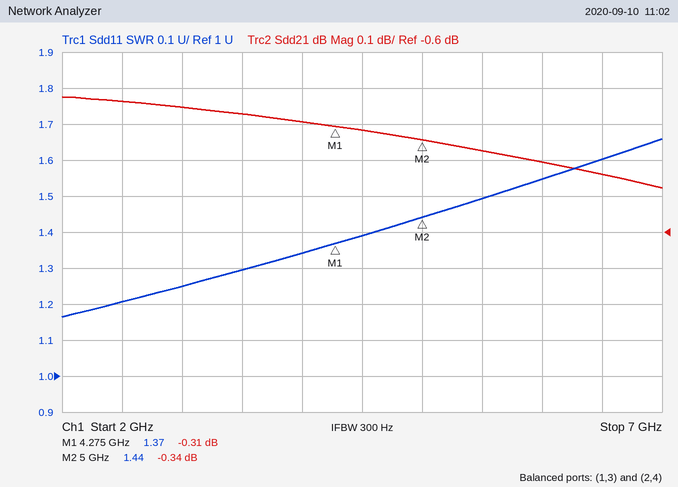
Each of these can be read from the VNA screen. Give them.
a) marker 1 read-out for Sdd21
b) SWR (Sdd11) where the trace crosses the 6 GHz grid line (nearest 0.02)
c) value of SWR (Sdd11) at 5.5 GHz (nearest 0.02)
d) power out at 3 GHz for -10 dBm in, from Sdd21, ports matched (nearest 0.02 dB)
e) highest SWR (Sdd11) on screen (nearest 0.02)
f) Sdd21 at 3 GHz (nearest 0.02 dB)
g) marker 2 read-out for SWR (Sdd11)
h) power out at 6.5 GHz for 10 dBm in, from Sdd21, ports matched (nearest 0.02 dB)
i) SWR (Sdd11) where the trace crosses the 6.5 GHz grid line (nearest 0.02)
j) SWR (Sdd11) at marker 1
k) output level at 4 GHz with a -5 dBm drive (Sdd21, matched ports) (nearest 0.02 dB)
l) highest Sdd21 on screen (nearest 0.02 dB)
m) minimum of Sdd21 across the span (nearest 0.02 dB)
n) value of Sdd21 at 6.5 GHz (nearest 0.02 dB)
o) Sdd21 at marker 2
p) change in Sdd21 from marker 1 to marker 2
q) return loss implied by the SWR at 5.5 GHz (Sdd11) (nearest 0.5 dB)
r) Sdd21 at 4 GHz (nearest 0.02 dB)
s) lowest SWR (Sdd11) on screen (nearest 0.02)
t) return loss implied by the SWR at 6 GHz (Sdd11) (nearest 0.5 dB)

-0.31 dB
1.54
1.50
-10.26 dBm
1.66
-0.26 dB
1.44
9.56 dBm
1.60
1.37
-5.30 dBm
-0.22 dB
-0.48 dB
-0.44 dB
-0.34 dB
-0.03 dB
14.0 dB
-0.30 dB
1.16
13.5 dB
